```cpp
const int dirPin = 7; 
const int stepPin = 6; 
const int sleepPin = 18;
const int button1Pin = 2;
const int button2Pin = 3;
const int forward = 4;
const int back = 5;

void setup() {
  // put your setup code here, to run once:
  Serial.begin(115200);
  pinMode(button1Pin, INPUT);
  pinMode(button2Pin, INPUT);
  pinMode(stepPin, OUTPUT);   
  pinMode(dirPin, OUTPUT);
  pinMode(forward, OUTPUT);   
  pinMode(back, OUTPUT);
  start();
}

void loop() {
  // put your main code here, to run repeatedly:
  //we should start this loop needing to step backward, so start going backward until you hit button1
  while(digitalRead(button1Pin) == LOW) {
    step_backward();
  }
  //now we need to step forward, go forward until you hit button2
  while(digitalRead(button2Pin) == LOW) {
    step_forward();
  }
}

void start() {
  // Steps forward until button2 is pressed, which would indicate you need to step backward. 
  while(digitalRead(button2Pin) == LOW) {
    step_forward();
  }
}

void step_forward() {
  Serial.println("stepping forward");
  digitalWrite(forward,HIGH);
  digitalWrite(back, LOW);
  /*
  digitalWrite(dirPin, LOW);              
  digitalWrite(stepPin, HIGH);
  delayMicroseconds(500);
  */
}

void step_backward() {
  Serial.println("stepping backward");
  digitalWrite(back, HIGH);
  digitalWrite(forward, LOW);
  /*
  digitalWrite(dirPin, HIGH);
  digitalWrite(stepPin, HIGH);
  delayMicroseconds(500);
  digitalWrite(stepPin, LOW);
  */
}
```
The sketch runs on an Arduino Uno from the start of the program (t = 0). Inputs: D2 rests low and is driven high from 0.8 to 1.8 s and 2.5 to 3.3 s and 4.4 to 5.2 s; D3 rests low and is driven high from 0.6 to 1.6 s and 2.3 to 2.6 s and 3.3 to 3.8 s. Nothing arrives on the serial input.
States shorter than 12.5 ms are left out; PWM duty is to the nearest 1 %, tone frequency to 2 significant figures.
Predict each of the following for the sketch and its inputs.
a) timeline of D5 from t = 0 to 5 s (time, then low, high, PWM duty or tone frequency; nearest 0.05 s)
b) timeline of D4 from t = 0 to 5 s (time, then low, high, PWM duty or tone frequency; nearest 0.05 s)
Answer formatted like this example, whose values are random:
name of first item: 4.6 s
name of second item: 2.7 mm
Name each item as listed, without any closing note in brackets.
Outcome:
timeline of D5 from t = 0 to 5 s: 0 s low; 0.6 s high; 1.6 s low; 2.3 s high; 2.6 s low; 3.3 s high; 4.4 s low
timeline of D4 from t = 0 to 5 s: 0 s high; 0.6 s low; 1.6 s high; 2.3 s low; 2.6 s high; 3.3 s low; 4.4 s high
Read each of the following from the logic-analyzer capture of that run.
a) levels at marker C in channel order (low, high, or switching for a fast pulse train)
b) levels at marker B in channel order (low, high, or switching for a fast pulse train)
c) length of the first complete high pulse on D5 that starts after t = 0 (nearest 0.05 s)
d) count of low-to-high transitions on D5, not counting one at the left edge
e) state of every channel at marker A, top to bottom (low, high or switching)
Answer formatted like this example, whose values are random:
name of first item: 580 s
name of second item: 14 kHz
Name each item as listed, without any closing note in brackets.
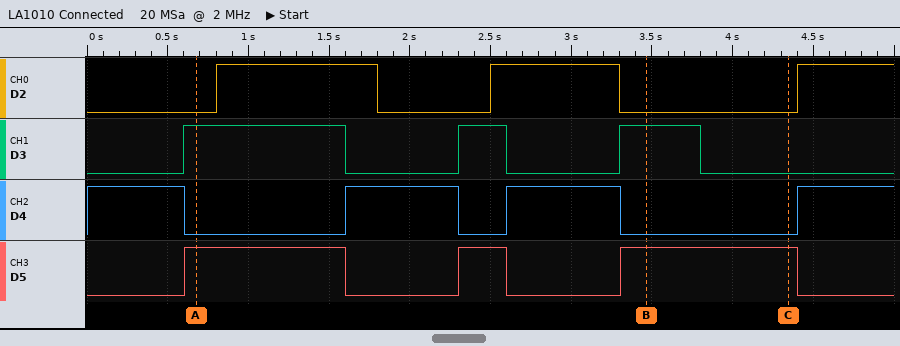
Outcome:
levels at marker C in channel order: D2 low, D3 low, D4 low, D5 high
levels at marker B in channel order: D2 low, D3 high, D4 low, D5 high
length of the first complete high pulse on D5 that starts after t = 0: 1.00 s
count of low-to-high transitions on D5, not counting one at the left edge: 3
state of every channel at marker A, top to bottom: D2 low, D3 high, D4 low, D5 high
